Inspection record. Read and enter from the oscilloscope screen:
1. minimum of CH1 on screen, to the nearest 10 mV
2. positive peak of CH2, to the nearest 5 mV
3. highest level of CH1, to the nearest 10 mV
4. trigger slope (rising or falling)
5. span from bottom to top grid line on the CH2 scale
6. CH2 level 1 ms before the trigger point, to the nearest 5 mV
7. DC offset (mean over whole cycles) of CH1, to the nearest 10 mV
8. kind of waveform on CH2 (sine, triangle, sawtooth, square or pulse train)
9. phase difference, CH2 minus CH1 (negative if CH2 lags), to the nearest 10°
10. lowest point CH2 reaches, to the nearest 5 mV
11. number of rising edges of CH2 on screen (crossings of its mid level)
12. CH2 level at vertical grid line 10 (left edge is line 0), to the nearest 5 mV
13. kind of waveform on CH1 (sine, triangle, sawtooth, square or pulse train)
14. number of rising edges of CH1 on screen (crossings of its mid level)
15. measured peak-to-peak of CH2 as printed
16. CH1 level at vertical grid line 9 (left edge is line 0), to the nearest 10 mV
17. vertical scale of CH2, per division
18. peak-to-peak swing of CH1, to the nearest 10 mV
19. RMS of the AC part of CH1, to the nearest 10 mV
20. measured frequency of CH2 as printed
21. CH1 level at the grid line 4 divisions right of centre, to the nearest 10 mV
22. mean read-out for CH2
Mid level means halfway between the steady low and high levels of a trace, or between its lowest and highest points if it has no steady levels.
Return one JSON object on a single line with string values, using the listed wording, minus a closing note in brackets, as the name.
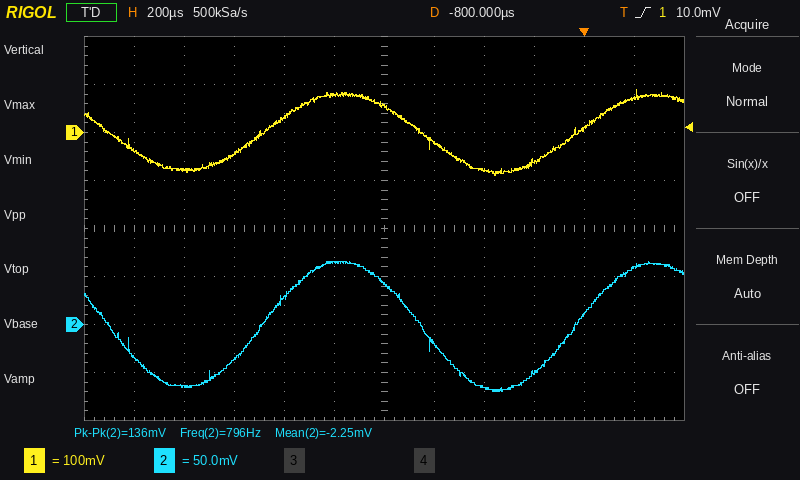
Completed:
{"minimum of CH1 on screen, to the nearest 10 mV": "-90 mV", "positive peak of CH2, to the nearest 5 mV": "65 mV", "highest level of CH1, to the nearest 10 mV": "90 mV", "trigger slope": "rising", "span from bottom to top grid line on the CH2 scale": "400 mV", "CH2 level 1 ms before the trigger point, to the nearest 5 mV": "65 mV", "DC offset (mean over whole cycles) of CH1, to the nearest 10 mV": "0 mV", "kind of waveform on CH2": "sine", "phase difference, CH2 minus CH1 (negative if CH2 lags), to the nearest 10°": "0°", "lowest point CH2 reaches, to the nearest 5 mV": "-70 mV", "number of rising edges of CH2 on screen": "2", "CH2 level at vertical grid line 10 (left edge is line 0), to the nearest 5 mV": "10 mV", "kind of waveform on CH1": "sine", "number of rising edges of CH1 on screen": "2", "measured peak-to-peak of CH2 as printed": "136 mV", "CH1 level at vertical grid line 9 (left edge is line 0), to the nearest 10 mV": "-60 mV", "vertical scale of CH2, per division": "50 mV", "peak-to-peak swing of CH1, to the nearest 10 mV": "180 mV", "RMS of the AC part of CH1, to the nearest 10 mV": "60 mV", "measured frequency of CH2 as printed": "796 Hz", "CH1 level at the grid line 4 divisions right of centre, to the nearest 10 mV": "10 mV", "mean read-out for CH2": "-2.25 mV"}
